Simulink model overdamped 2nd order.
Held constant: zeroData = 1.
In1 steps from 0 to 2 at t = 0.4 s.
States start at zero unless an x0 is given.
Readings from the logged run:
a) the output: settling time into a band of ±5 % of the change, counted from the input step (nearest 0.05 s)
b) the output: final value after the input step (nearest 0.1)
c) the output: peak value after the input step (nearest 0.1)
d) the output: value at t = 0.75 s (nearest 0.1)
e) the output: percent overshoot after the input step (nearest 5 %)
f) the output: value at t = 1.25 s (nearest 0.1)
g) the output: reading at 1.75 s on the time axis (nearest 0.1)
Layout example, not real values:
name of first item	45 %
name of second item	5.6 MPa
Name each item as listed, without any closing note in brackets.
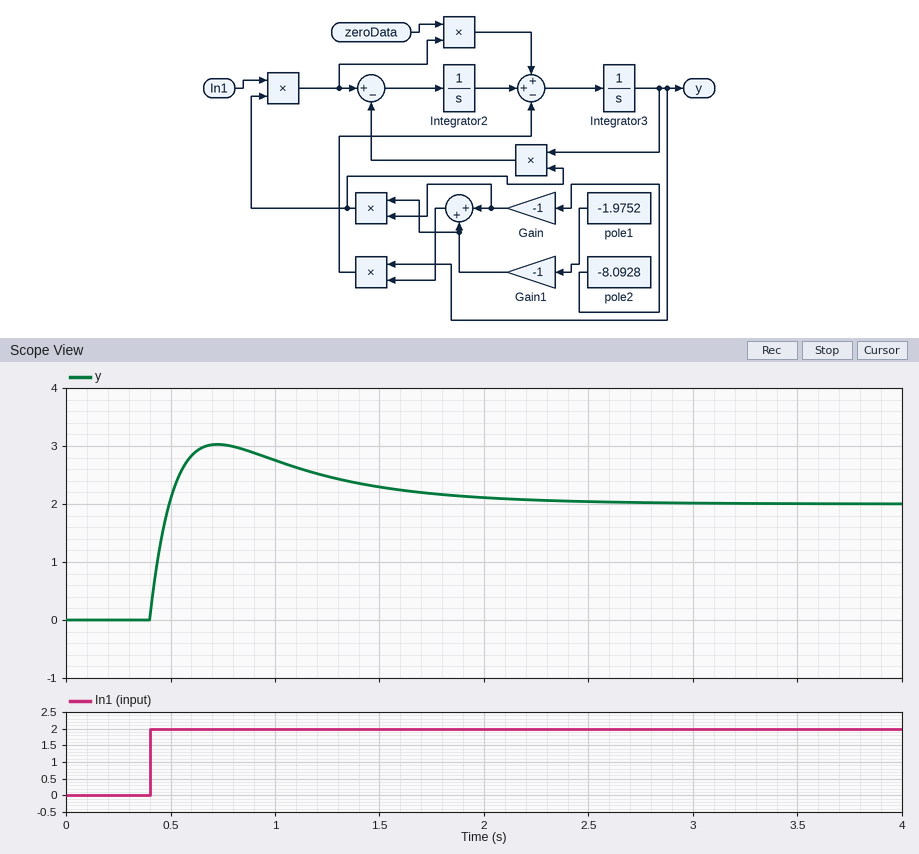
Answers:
the output: settling time into a band of ±5 % of the change, counted from the input step	1.65 s
the output: final value after the input step	2.0
the output: peak value after the input step	3.0
the output: value at t = 0.75 s	3.0
the output: percent overshoot after the input step	50 %
the output: value at t = 1.25 s	2.5
the output: reading at 1.75 s on the time axis	2.2
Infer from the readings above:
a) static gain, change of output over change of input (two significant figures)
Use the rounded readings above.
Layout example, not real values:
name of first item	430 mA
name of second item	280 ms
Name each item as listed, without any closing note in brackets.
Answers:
static gain, change of output over change of input	1.0
